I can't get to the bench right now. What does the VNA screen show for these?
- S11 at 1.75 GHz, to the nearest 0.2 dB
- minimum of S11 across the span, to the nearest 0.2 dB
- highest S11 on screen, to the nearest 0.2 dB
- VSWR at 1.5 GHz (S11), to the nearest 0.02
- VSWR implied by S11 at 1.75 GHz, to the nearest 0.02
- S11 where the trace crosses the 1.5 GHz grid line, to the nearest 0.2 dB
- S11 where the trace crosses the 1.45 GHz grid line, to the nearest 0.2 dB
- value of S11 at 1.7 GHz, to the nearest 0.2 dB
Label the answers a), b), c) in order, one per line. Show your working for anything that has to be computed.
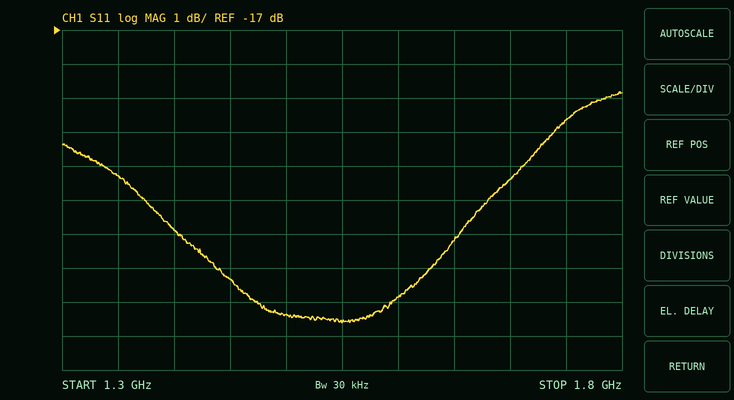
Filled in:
a) -19.6 dB
b) -25.6 dB
c) -18.8 dB
d) |Γ| = 10^(-25.4/20) = 0.0537; VSWR = (1 + 0.0537)/(1 − 0.0537) ≈ 1.11, so 1.12 to the nearest 0.02
e) |Γ| = 10^(-19.6/20) = 0.1047; VSWR = (1 + 0.1047)/(1 − 0.1047) ≈ 1.23, so 1.24 to the nearest 0.02
f) -25.4 dB
g) -24.4 dB
h) -21.4 dB
